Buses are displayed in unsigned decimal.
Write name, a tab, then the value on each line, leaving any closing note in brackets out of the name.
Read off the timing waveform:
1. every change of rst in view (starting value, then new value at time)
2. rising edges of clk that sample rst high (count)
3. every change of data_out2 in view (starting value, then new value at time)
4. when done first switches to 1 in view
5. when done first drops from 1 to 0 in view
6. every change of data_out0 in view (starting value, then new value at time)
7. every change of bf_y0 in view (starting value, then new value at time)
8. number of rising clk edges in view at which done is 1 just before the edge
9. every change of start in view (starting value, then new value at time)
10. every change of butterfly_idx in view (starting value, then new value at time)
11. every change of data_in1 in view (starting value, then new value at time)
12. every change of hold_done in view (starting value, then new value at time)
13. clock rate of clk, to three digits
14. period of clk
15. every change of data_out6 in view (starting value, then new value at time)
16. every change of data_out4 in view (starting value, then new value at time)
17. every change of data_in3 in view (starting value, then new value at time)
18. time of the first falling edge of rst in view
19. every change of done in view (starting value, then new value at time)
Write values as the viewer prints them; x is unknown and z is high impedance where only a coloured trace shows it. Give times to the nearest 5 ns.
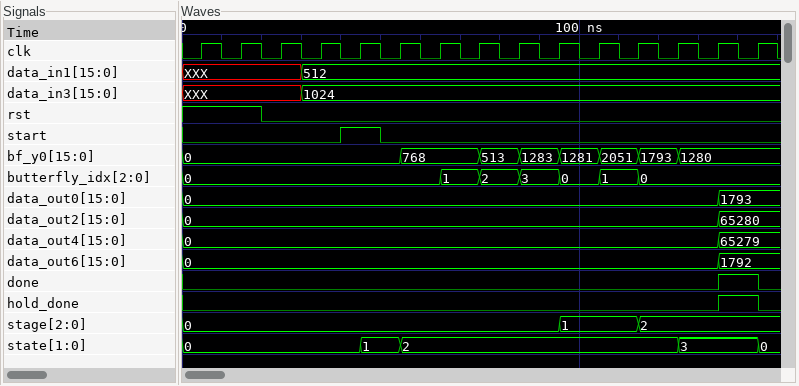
every change of rst in view	1, 0 at 20 ns
rising edges of clk that sample rst high	2
every change of data_out2 in view	0, 65280 at 135 ns
when done first switches to 1 in view	135 ns
when done first drops from 1 to 0 in view	145 ns
every change of data_out0 in view	0, 1793 at 135 ns
every change of bf_y0 in view	0, 768 at 55 ns, 513 at 75 ns, 1283 at 85 ns, 1281 at 95 ns, 2051 at 105 ns, 1793 at 115 ns, 1280 at 125 ns
number of rising clk edges in view at which done is 1 just before the edge	1
every change of start in view	0, 1 at 40 ns, 0 at 50 ns
every change of butterfly_idx in view	0, 1 at 65 ns, 2 at 75 ns, 3 at 85 ns, 0 at 95 ns, 1 at 105 ns, 0 at 115 ns
every change of data_in1 in view	XXX, 512 at 30 ns
every change of hold_done in view	0, 1 at 135 ns, 0 at 145 ns
clock rate of clk, to three digits	100 MHz
period of clk	10 ns
every change of data_out6 in view	0, 1792 at 135 ns
every change of data_out4 in view	0, 65279 at 135 ns
every change of data_in3 in view	XXX, 1024 at 30 ns
time of the first falling edge of rst in view	20 ns
every change of done in view	0, 1 at 135 ns, 0 at 145 ns
